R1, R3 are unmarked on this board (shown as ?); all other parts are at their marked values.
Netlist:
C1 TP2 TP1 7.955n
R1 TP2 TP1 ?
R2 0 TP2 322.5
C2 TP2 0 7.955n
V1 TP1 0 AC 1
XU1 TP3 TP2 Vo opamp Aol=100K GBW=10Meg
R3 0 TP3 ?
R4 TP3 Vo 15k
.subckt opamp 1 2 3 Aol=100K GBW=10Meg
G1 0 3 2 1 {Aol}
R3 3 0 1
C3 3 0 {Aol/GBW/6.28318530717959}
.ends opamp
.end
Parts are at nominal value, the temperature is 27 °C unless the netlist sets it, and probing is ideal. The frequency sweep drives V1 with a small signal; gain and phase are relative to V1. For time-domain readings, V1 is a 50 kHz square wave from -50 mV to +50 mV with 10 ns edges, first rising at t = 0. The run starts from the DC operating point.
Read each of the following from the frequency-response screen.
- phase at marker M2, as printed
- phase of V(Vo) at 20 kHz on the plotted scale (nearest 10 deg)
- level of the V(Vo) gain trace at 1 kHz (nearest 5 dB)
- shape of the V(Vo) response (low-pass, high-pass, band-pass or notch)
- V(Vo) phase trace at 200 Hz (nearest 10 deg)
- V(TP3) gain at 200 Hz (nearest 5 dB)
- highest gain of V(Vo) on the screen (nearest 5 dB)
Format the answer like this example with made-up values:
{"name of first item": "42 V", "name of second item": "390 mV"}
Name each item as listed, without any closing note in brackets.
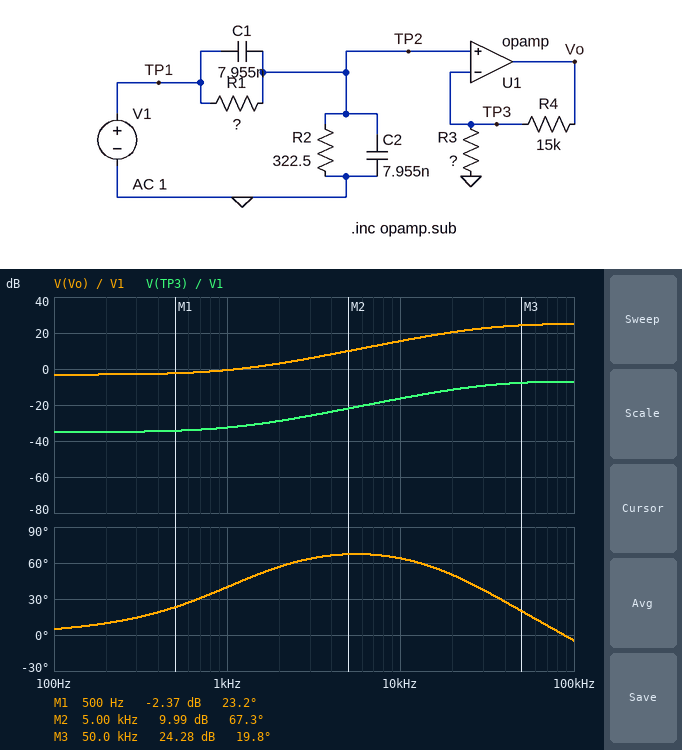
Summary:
{"phase at marker M2, as printed": "67.3 deg", "phase of V(Vo) at 20 kHz on the plotted scale": "50 deg", "level of the V(Vo) gain trace at 1 kHz": "0 dB", "shape of the V(Vo) response": "high-pass", "V(Vo) phase trace at 200 Hz": "10 deg", "V(TP3) gain at 200 Hz": "-35 dB", "highest gain of V(Vo) on the screen": "25 dB"}
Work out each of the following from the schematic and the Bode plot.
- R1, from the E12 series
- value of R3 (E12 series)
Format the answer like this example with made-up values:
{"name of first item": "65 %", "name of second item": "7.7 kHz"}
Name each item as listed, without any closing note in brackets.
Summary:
{"R1, from the E12 series": "18 kΩ", "value of R3": "390 Ω"}
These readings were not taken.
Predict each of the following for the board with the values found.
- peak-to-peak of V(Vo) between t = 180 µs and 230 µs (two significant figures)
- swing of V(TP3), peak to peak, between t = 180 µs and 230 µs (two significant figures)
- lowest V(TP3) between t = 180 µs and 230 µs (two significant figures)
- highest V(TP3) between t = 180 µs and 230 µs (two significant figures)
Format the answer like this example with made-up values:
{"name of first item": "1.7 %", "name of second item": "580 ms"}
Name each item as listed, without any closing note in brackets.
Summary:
{"peak-to-peak of V(Vo) between t = 180 µs and 230 µs": "2.5 V", "swing of V(TP3), peak to peak, between t = 180 µs and 230 µs": "63 mV", "lowest V(TP3) between t = 180 µs and 230 µs": "-32 mV", "highest V(TP3) between t = 180 µs and 230 µs": "32 mV"}
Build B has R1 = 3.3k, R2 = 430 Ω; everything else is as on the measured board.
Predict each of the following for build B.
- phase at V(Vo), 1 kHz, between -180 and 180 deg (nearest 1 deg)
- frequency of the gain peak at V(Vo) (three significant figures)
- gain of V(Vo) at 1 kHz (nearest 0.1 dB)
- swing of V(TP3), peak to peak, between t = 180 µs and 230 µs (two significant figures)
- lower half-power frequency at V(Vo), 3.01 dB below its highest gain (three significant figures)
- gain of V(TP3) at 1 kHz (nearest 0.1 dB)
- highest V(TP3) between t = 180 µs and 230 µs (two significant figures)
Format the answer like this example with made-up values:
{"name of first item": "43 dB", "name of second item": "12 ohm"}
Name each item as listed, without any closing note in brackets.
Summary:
{"phase at V(Vo), 1 kHz, between -180 and 180 deg": "7 deg", "frequency of the gain peak at V(Vo)": "80.3 kHz", "gain of V(Vo) at 1 kHz": "13.3 dB", "swing of V(TP3), peak to peak, between t = 180 µs and 230 µs": "59 mV", "lower half-power frequency at V(Vo), 3.01 dB below its highest gain": "20.7 kHz", "gain of V(TP3) at 1 kHz": "-18.7 dB", "highest V(TP3) between t = 180 µs and 230 µs": "29 mV"}
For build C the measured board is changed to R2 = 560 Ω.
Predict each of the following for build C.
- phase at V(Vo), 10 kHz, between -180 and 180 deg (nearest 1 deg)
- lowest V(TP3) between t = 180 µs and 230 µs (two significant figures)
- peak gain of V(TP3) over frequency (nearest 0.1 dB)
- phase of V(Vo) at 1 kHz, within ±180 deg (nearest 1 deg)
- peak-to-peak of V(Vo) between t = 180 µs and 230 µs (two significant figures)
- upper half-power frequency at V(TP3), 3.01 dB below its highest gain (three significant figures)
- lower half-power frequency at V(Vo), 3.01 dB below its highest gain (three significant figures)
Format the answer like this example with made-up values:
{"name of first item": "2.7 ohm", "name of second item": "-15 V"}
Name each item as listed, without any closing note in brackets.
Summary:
{"phase at V(Vo), 10 kHz, between -180 and 180 deg": "53 deg", "lowest V(TP3) between t = 180 µs and 230 µs": "-30 mV", "peak gain of V(TP3) over frequency": "-6.6 dB", "phase of V(Vo) at 1 kHz, within ±180 deg": "39 deg", "peak-to-peak of V(Vo) between t = 180 µs and 230 µs": "2.4 V", "upper half-power frequency at V(TP3), 3.01 dB below its highest gain": "288 kHz", "lower half-power frequency at V(Vo), 3.01 dB below its highest gain": "16.1 kHz"}
